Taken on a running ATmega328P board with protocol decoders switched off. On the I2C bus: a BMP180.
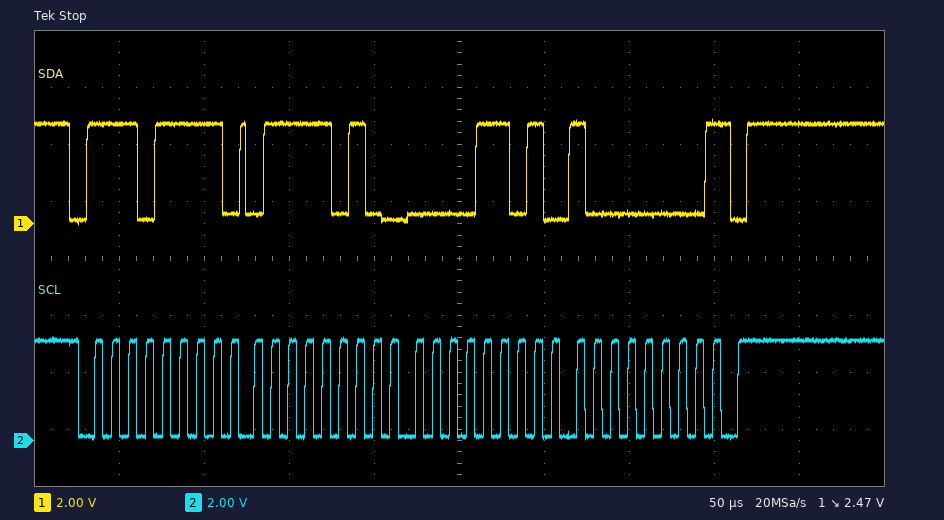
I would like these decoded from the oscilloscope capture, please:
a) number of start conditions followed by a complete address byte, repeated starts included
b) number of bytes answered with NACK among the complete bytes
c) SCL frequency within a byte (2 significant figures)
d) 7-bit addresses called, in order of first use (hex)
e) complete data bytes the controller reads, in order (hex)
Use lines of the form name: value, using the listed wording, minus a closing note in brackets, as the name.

number of start conditions followed by a complete address byte, repeated starts included: 1
number of bytes answered with NACK among the complete bytes: 1
SCL frequency within a byte: 100 kHz
7-bit addresses called, in order of first use: 0x77
complete data bytes the controller reads, in order: 7A 0D 80
